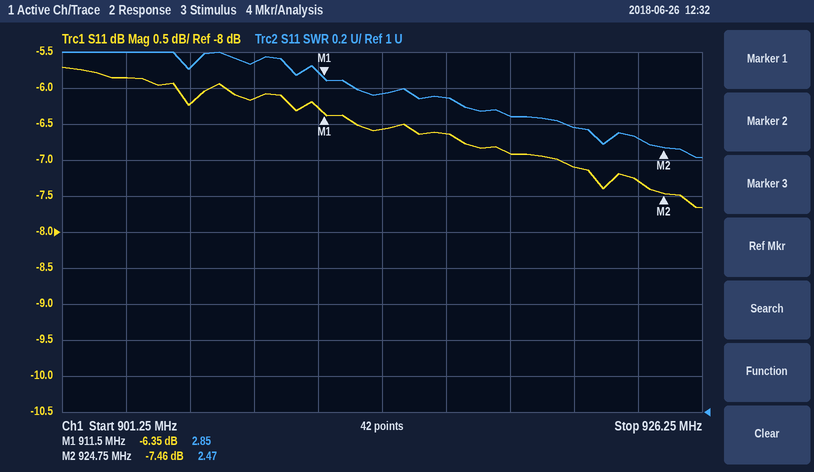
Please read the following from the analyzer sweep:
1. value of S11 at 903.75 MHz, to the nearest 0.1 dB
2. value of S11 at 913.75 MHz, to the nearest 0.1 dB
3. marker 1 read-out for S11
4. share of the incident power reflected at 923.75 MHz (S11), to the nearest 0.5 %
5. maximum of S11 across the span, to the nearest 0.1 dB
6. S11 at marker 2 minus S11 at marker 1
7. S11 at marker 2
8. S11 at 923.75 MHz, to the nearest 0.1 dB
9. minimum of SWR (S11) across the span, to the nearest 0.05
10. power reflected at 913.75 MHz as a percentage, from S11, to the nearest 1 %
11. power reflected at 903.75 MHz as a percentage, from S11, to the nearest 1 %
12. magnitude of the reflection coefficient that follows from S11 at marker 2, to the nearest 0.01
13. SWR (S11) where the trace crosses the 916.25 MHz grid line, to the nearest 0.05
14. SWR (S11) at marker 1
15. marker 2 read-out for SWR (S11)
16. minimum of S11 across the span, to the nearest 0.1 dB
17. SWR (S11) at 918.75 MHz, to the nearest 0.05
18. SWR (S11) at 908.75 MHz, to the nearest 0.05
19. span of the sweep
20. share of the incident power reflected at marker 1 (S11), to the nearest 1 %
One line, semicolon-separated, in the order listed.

-5.9 dB; -6.6 dB; -6.35 dB; 18.5 %; -5.7 dB; -1.11 dB; -7.46 dB; -7.3 dB; 2.40; 22 %; 26 %; 0.42; 2.75; 2.85; 2.47; -7.7 dB; 2.65; 2.95; 25 MHz; 23 %
